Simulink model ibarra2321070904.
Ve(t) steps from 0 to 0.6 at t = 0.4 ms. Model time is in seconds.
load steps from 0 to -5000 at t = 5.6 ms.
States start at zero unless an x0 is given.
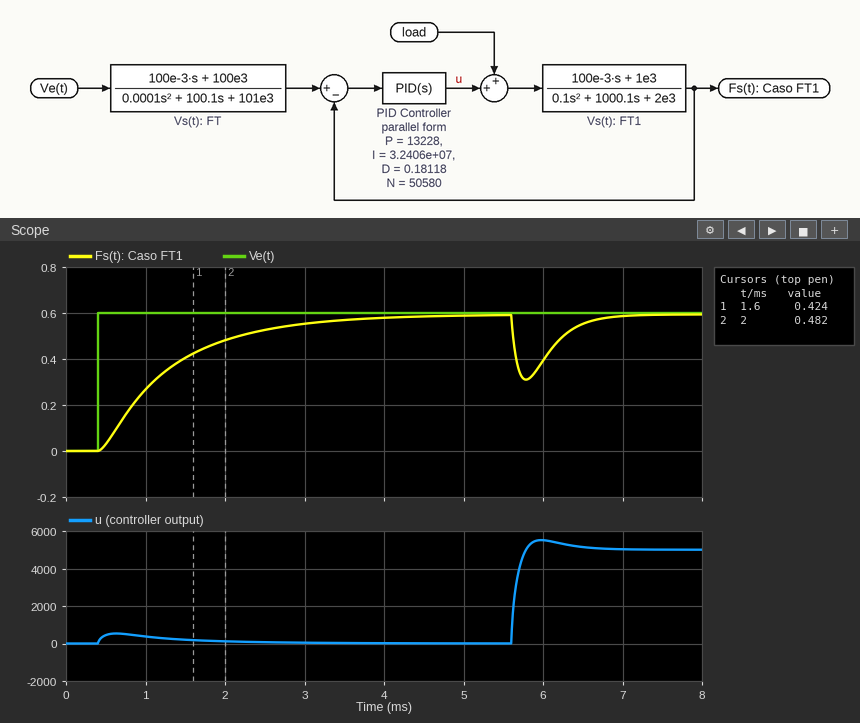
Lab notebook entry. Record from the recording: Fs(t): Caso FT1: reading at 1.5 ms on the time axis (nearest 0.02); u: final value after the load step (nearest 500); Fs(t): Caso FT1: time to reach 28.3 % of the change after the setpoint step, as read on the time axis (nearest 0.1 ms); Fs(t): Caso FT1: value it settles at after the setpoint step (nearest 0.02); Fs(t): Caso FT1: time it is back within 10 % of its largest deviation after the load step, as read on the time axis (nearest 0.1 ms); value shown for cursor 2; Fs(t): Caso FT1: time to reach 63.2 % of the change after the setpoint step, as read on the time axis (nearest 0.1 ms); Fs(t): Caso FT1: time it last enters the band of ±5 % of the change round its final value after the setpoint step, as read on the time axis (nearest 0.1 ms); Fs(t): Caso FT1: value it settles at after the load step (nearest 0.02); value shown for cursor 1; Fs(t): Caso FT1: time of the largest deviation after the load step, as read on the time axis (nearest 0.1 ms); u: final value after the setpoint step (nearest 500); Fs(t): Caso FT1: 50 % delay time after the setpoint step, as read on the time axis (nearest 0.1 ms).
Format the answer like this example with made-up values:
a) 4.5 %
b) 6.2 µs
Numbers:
a) 0.40
b) 5000
c) 0.8 ms
d) 0.60
e) 6.6 ms
f) 0.482
g) 1.4 ms
h) 3.3 ms
i) 0.60
j) 0.424
k) 5.8 ms
l) 0
m) 1.1 ms
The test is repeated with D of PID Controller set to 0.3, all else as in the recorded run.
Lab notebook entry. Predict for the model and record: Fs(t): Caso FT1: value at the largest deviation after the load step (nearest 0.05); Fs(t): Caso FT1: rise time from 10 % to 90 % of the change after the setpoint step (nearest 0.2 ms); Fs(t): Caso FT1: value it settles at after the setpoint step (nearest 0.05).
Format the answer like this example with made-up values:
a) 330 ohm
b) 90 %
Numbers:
a) 0.30
b) 2.0 ms
c) 0.60
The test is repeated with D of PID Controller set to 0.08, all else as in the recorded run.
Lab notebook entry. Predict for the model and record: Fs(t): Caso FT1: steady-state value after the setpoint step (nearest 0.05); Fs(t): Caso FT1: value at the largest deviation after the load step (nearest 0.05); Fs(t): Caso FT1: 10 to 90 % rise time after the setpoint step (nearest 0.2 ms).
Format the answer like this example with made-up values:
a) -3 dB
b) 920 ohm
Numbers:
a) 0.60
b) 0.30
c) 2.0 ms
